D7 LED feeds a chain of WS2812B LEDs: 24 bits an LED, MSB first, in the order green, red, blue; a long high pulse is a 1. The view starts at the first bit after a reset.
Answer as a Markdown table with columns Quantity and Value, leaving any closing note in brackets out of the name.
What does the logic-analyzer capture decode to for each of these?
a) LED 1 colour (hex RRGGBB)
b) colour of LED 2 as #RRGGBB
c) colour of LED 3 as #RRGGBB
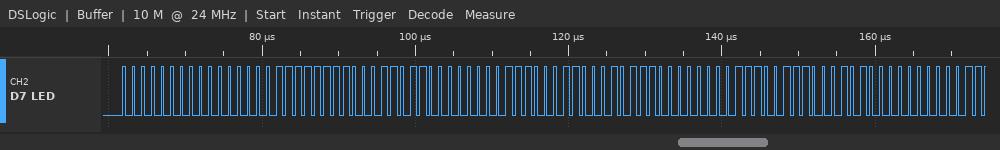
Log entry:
| Quantity | Value |
|---|---|
| LED 1 colour | #0000FF |
| colour of LED 2 as #RRGGBB | #001BE3 |
| colour of LED 3 as #RRGGBB | #0017E7 |
